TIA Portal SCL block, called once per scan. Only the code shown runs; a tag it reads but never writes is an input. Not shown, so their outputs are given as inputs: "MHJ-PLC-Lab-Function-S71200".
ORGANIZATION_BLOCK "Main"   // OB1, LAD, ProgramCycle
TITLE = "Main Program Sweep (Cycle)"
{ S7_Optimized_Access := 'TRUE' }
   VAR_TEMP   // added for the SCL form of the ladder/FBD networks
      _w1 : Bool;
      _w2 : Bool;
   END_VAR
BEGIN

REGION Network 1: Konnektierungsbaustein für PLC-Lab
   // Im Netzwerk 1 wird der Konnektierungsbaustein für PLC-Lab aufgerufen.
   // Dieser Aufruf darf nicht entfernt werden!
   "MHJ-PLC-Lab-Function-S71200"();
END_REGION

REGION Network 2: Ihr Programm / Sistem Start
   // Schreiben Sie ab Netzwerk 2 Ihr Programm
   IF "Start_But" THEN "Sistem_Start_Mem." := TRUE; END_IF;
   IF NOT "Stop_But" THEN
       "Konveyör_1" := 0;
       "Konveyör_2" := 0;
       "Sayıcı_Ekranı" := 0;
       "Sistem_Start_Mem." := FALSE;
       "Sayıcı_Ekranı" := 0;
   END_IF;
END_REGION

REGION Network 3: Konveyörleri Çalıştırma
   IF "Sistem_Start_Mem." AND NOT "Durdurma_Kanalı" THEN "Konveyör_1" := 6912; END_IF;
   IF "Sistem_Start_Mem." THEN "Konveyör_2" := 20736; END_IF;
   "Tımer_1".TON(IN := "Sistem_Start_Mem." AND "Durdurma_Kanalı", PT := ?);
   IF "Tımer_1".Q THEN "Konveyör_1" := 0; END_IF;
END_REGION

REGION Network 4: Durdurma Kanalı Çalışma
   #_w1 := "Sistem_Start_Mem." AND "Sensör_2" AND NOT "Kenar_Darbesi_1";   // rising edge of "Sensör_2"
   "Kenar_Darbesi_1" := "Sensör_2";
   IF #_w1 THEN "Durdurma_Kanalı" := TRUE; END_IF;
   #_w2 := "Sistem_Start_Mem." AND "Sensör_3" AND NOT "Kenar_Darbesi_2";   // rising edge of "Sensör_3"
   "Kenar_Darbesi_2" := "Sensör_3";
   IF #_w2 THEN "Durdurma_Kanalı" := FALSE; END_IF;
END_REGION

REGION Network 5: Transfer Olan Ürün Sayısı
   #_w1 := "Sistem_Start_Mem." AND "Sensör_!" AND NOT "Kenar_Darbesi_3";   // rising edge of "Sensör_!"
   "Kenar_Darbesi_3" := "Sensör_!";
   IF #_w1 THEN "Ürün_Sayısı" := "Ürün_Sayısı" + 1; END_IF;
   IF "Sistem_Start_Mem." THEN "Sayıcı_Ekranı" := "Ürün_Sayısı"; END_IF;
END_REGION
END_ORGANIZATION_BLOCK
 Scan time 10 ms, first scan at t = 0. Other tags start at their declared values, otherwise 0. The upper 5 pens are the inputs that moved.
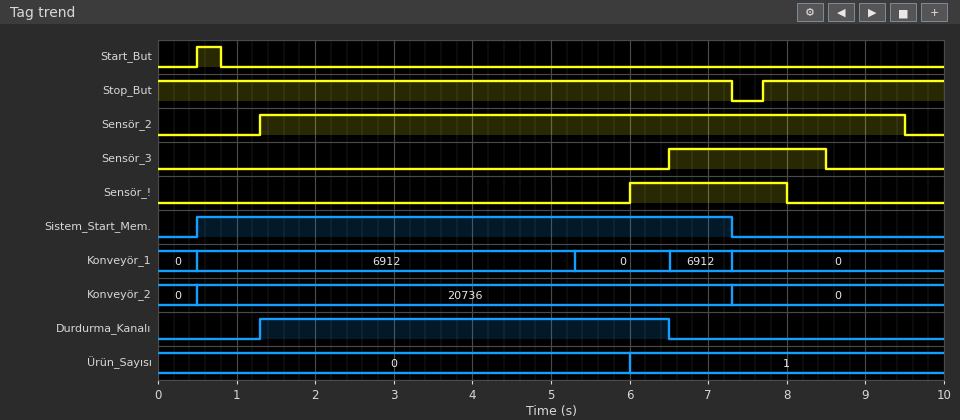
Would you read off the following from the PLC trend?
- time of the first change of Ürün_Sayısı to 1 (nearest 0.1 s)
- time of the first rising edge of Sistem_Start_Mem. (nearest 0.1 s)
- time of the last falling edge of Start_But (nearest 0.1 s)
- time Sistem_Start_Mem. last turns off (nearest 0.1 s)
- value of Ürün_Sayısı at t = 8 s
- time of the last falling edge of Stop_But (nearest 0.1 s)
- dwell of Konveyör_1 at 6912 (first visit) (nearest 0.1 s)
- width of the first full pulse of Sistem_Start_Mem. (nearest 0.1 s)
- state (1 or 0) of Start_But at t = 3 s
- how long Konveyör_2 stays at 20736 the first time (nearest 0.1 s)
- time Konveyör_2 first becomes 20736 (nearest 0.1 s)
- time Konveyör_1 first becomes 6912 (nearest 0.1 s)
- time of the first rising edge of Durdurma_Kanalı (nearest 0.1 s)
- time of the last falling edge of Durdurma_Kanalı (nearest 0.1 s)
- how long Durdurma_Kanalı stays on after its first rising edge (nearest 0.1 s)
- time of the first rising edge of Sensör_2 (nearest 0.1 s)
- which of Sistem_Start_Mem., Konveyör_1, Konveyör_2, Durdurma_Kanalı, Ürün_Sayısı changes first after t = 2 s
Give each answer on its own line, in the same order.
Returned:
6.0 s
0.5 s
0.8 s
7.3 s
1
7.3 s
4.8 s
6.8 s
0
6.8 s
0.5 s
0.5 s
1.3 s
6.5 s
5.2 s
1.3 s
Konveyör_1
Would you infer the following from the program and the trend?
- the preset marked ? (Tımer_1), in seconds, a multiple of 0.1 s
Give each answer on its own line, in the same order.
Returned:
4.0 s
